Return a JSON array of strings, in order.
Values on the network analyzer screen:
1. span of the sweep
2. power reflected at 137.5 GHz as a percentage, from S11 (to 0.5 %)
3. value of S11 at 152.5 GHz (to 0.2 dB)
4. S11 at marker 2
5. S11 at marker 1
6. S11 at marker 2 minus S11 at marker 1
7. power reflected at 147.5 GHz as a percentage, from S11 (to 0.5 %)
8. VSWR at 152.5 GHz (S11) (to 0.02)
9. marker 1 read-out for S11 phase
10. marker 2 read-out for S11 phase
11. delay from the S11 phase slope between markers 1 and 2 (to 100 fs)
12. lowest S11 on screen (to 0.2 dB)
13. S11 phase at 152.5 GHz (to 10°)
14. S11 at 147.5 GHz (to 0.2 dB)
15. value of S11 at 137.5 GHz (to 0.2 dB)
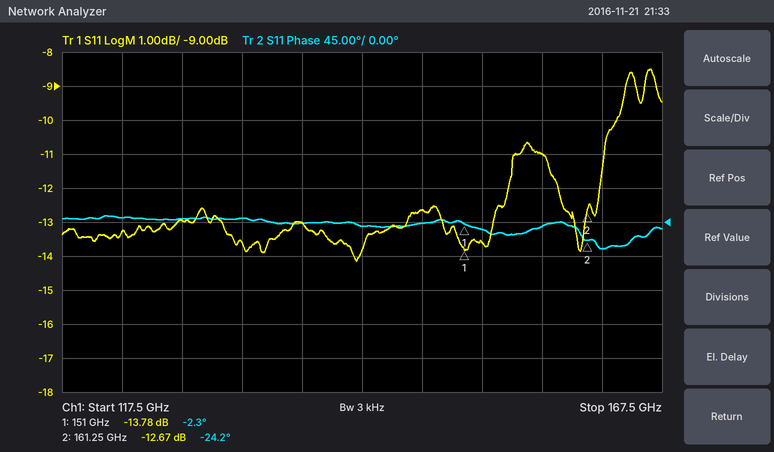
["50 GHz", "5.0 %", "-13.6 dB", "-12.67 dB", "-13.78 dB", "1.11 dB", "5.5 %", "1.52", "-2.3°", "-24.2°", "5.9 ps", "-14.2 dB", "-10°", "-12.6 dB", "-13.0 dB"]
